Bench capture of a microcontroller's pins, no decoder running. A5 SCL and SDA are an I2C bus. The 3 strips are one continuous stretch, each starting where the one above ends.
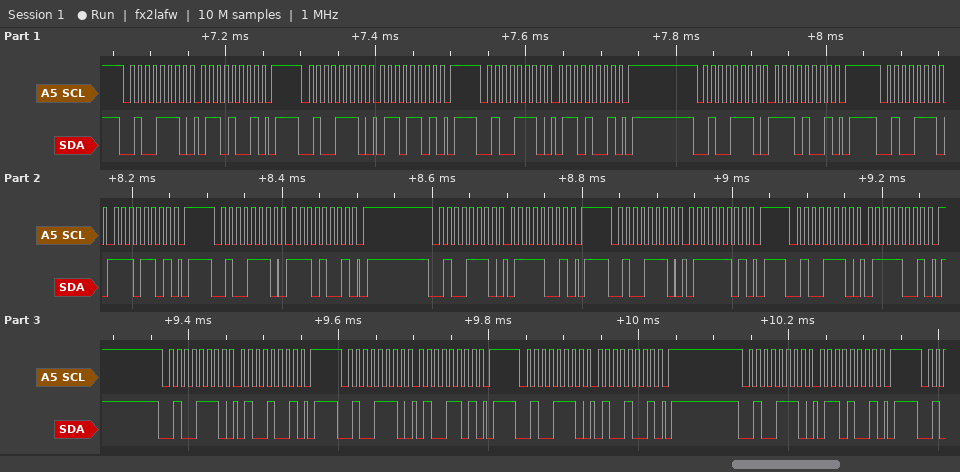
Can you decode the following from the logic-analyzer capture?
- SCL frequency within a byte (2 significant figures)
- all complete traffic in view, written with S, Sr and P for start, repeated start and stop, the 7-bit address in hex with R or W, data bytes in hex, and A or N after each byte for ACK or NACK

100 kHz
S 27W A 69 A P S 27W A 6D A P S 27W A 69 A P S 27W A E9 A P S 27W A ED A P S 27W A E9 A P S 27W A 79 A P S 27W A 7D A P S 27W A 79 A P S 27W A 49 A P S 27W A 4D A P S 27W A 49 A P S 27W A 69 A P
